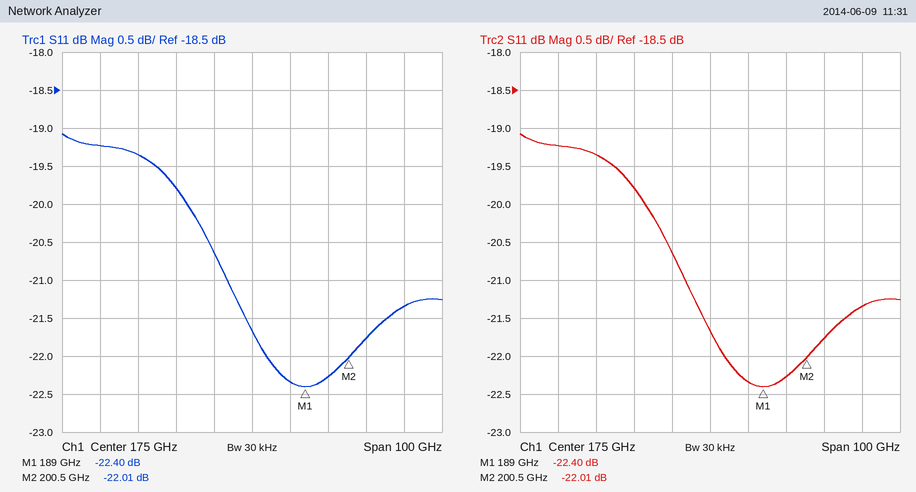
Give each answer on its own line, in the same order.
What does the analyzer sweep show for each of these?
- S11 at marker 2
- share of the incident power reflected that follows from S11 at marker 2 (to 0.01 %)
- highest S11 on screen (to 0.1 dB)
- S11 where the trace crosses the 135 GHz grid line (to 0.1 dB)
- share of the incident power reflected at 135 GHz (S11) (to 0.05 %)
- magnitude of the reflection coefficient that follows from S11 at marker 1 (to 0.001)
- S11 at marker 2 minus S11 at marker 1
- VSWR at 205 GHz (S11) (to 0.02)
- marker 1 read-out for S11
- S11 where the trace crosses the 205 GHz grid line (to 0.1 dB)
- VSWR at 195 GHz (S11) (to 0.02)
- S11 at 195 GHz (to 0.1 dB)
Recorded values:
-22.01 dB
0.63 %
-19.1 dB
-19.2 dB
1.20 %
0.076
0.39 dB
1.18
-22.40 dB
-21.8 dB
1.16
-22.3 dB
